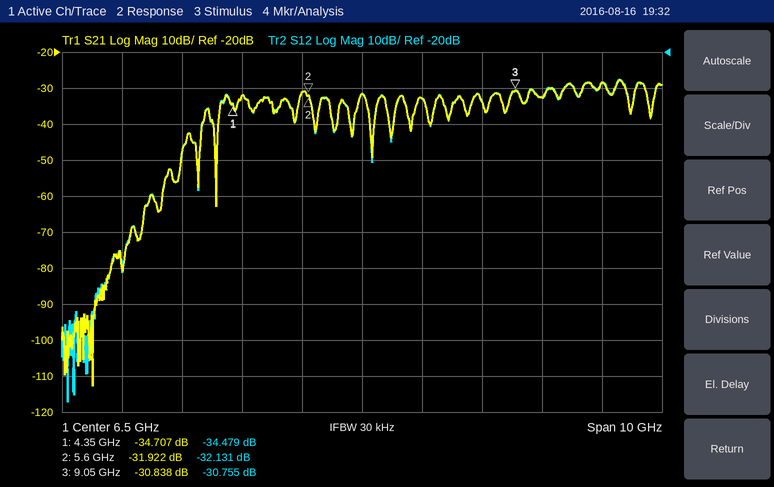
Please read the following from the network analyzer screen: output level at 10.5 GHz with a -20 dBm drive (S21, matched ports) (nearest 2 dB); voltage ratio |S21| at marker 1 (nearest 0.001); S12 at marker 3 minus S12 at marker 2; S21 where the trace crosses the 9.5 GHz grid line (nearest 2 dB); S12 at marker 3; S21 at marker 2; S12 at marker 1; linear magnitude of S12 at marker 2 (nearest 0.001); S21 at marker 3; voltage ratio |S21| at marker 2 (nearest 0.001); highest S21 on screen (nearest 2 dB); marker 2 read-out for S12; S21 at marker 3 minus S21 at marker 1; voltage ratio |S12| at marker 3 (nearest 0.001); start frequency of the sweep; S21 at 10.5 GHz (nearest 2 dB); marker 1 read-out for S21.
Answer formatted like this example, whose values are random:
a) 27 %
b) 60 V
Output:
a) -48 dBm
b) 0.018
c) 1.376 dB
d) -32 dB
e) -30.755 dB
f) -31.922 dB
g) -34.479 dB
h) 0.025
i) -30.838 dB
j) 0.025
k) -28 dB
l) -32.131 dB
m) 3.869 dB
n) 0.029
o) 1.5 GHz
p) -28 dB
q) -34.707 dB
